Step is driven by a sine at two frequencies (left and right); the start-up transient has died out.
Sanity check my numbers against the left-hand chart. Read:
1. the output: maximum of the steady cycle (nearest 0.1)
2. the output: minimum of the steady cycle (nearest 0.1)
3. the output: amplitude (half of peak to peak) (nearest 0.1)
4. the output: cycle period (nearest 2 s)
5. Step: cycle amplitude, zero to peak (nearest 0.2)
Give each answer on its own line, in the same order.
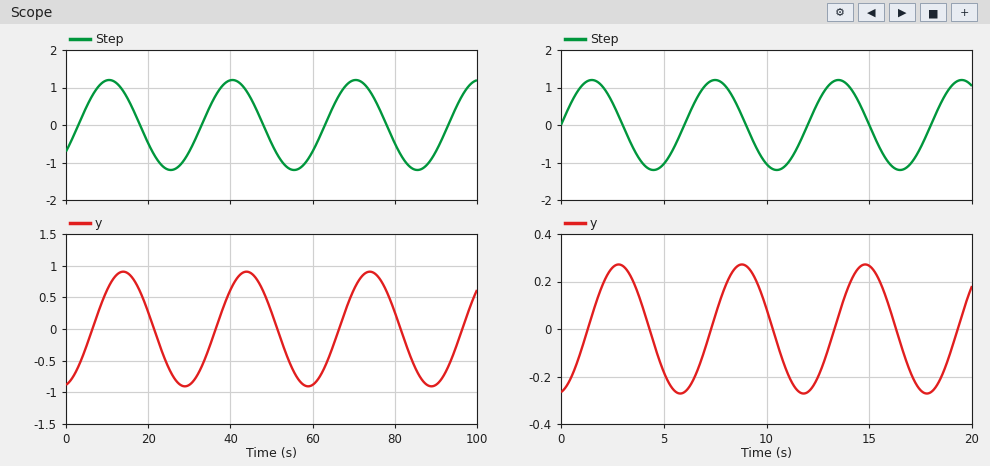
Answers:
0.9
-0.9
0.9
30 s
1.2
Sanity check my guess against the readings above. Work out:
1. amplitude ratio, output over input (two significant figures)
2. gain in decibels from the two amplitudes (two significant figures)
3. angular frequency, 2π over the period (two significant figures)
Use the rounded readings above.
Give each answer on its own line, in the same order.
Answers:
0.75
-2.5 dB
0.21 rad/s
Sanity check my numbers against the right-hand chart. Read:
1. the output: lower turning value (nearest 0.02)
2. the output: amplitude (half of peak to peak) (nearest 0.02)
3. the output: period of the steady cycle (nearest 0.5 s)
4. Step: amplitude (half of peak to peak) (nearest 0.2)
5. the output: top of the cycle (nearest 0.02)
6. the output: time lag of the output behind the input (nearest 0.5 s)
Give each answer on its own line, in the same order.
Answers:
-0.28
0.28
6.0 s
1.2
0.28
1.5 s
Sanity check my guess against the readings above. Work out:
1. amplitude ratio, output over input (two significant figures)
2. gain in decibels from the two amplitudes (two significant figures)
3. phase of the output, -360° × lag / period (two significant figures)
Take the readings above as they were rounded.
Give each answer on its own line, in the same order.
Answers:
0.23
-13 dB
-90°
